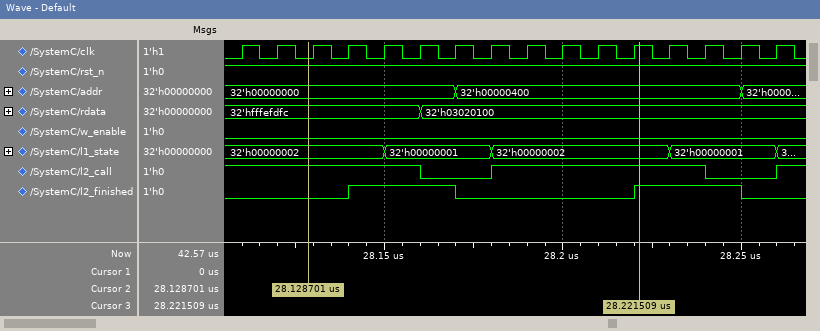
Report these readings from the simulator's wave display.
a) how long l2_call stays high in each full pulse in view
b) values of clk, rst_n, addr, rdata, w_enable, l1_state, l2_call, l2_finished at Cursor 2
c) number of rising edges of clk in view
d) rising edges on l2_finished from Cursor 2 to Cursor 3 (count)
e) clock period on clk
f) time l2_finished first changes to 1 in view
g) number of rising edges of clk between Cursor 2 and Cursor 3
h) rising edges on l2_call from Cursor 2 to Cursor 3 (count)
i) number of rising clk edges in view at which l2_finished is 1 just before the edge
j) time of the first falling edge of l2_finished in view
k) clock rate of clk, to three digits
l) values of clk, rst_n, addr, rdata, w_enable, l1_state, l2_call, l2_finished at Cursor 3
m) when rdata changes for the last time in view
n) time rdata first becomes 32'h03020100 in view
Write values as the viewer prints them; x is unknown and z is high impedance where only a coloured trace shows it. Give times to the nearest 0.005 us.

0.06 us
clk=0, rst_n=1, addr=32'h00000000, rdata=32'hfffefdfc, w_enable=0, l1_state=32'h00000002, l2_call=1, l2_finished=0
16
2
0.01 us
28.14 us
10
1
6
28.17 us
100 MHz
clk=1, rst_n=1, addr=32'h00000400, rdata=32'h03020100, w_enable=0, l1_state=32'h00000002, l2_call=1, l2_finished=1
28.16 us
28.16 us
